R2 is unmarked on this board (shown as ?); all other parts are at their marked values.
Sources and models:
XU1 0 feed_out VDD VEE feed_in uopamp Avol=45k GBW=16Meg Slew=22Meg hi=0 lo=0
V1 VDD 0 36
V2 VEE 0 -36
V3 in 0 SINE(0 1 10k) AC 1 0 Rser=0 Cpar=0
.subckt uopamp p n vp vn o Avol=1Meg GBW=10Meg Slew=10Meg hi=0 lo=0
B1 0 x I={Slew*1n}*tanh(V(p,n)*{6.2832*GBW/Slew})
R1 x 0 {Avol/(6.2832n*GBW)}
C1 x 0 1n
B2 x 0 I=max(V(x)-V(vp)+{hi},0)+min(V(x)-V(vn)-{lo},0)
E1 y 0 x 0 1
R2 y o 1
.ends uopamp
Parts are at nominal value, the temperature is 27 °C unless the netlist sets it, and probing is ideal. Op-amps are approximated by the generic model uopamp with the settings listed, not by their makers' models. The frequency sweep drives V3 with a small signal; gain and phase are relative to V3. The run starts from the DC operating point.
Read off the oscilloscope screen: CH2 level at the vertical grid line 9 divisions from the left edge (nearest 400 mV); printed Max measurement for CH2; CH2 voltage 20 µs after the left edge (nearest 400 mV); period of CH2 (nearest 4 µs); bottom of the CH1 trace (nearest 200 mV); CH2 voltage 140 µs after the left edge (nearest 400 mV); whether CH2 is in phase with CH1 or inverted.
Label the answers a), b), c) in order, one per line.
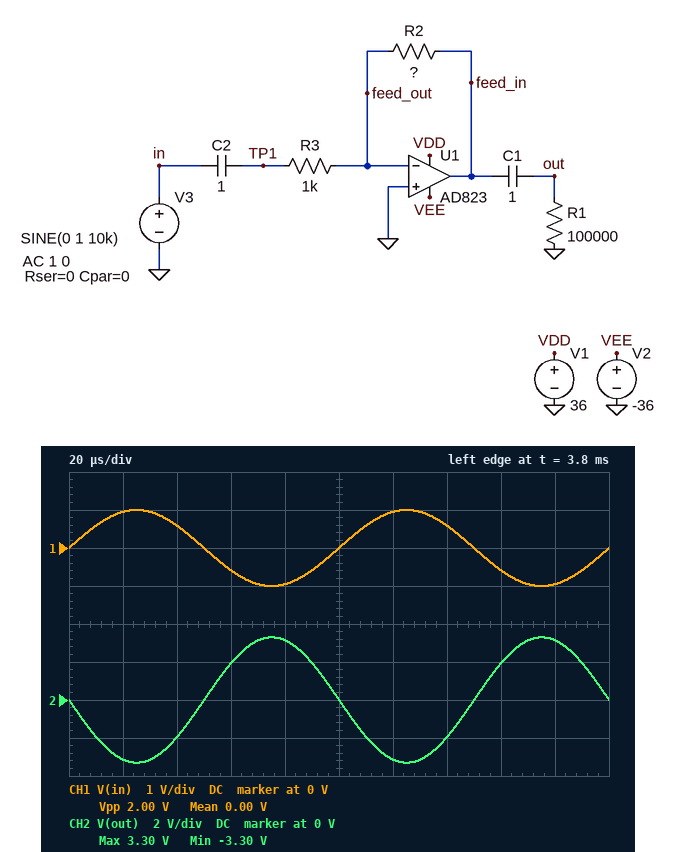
a) 3.2 V
b) 3.30 V
c) -3.2 V
d) 100 µs
e) -1.0 V
f) -2.0 V
g) inverted
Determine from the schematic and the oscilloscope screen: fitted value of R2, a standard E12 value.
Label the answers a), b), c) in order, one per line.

a) 3.3 kΩ
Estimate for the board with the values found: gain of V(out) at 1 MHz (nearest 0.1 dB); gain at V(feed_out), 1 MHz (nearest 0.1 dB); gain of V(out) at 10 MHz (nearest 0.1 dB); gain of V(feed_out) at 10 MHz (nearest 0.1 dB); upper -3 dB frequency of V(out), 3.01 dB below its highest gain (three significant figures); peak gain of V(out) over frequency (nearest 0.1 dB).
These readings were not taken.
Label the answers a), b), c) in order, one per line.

a) 10.1 dB
b) -14.0 dB
c) 1.2 dB
d) -2.9 dB
e) 3.72 MHz
f) 10.4 dB
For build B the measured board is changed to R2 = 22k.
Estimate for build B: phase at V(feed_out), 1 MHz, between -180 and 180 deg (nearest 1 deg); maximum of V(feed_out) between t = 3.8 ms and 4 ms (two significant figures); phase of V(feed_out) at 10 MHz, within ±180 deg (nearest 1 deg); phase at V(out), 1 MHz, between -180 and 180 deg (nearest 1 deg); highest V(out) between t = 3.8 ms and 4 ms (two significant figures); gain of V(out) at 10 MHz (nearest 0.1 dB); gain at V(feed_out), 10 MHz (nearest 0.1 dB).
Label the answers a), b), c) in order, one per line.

a) 35 deg
b) 14 mV
c) 4 deg
d) 125 deg
e) 22 V
f) 3.7 dB
g) -0.4 dB
